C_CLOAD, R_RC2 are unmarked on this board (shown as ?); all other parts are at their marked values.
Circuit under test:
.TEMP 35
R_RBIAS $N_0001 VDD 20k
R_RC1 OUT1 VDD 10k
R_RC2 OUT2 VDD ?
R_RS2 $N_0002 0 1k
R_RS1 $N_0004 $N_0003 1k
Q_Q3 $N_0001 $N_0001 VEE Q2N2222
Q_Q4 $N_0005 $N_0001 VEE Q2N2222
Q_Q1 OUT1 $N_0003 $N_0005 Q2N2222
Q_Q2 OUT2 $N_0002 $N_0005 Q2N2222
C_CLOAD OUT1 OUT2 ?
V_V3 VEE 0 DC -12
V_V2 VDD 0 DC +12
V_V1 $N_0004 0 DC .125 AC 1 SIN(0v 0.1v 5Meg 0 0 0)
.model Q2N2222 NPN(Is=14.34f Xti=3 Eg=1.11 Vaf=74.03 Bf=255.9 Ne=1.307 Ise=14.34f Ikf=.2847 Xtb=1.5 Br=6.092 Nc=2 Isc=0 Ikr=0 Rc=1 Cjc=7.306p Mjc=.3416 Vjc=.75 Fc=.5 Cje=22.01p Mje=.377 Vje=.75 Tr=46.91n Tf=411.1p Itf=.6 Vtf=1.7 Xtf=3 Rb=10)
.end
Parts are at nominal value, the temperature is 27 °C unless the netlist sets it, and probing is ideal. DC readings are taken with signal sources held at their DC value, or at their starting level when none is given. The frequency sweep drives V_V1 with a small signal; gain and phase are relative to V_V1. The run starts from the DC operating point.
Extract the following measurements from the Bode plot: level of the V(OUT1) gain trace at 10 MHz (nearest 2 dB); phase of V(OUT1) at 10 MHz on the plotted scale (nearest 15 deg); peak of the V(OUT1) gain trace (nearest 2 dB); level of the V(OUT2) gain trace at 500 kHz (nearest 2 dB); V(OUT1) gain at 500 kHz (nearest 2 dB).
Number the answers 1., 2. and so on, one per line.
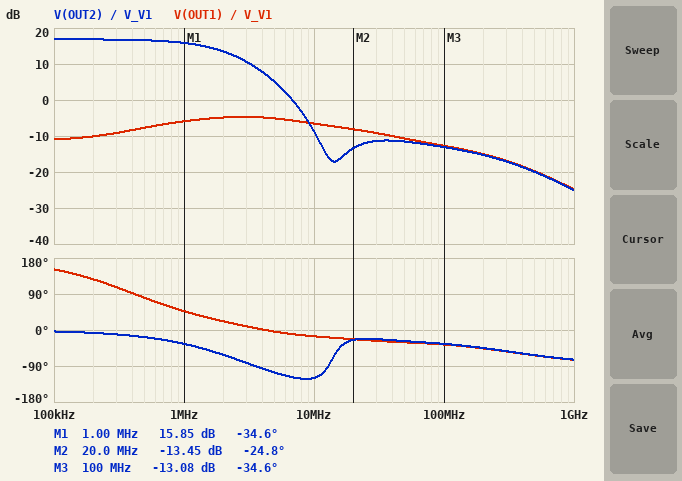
1. -6 dB
2. -15 deg
3. -4 dB
4. 16 dB
5. -8 dB
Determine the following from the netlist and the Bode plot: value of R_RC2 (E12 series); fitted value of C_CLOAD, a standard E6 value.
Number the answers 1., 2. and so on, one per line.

1. 12 kΩ
2. 3.3 pF
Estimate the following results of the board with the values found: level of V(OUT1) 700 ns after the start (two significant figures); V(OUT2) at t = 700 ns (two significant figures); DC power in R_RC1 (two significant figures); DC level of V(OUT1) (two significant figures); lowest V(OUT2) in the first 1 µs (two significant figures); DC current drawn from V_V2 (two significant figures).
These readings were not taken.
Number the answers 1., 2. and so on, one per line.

1. 4.9 V
2. 4.7 V
3. 16 mW
4. -480 mV
5. 4.0 V
6. 2.5 mA
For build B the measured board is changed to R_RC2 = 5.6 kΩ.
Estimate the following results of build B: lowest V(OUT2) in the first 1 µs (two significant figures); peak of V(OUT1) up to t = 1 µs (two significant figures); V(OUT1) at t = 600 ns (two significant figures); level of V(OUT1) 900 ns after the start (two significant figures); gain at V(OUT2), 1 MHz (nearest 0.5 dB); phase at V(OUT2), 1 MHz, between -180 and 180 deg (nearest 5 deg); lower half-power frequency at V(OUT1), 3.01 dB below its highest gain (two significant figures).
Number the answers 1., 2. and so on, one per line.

1. 8.0 V
2. 5.9 V
3. 5.8 V
4. 5.0 V
5. 10.0 dB
6. -20 deg
7. 590 kHz
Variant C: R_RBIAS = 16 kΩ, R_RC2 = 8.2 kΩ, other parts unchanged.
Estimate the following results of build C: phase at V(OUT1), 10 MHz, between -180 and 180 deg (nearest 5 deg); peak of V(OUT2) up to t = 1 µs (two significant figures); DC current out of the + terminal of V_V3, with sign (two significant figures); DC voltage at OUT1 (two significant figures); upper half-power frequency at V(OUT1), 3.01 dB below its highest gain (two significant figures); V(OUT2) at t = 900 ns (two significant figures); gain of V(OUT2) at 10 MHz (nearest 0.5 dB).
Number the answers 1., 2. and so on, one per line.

1. -5 deg
2. 5.9 V
3. -3.1 mA
4. -560 mV
5. 31 MHz
6. 5.7 V
7. 4.5 dB
